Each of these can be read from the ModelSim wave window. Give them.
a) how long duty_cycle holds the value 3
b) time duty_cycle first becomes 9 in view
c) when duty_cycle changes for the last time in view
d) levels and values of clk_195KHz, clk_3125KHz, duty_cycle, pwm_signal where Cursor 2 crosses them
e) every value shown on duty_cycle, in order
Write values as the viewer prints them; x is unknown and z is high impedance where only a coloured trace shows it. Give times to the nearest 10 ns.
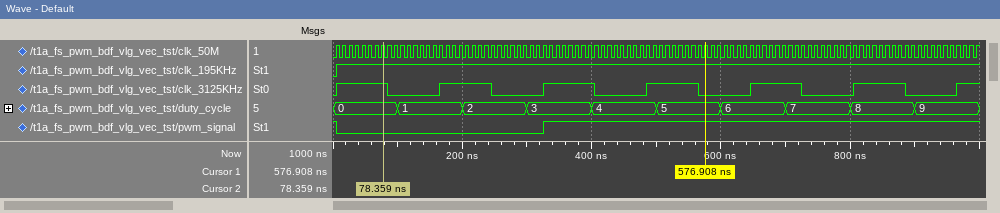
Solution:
100 ns
900 ns
900 ns
clk_195KHz=1, clk_3125KHz=1, duty_cycle=0, pwm_signal=0
0, 1, 2, 3, 4, 5, 6, 7, 8, 9
